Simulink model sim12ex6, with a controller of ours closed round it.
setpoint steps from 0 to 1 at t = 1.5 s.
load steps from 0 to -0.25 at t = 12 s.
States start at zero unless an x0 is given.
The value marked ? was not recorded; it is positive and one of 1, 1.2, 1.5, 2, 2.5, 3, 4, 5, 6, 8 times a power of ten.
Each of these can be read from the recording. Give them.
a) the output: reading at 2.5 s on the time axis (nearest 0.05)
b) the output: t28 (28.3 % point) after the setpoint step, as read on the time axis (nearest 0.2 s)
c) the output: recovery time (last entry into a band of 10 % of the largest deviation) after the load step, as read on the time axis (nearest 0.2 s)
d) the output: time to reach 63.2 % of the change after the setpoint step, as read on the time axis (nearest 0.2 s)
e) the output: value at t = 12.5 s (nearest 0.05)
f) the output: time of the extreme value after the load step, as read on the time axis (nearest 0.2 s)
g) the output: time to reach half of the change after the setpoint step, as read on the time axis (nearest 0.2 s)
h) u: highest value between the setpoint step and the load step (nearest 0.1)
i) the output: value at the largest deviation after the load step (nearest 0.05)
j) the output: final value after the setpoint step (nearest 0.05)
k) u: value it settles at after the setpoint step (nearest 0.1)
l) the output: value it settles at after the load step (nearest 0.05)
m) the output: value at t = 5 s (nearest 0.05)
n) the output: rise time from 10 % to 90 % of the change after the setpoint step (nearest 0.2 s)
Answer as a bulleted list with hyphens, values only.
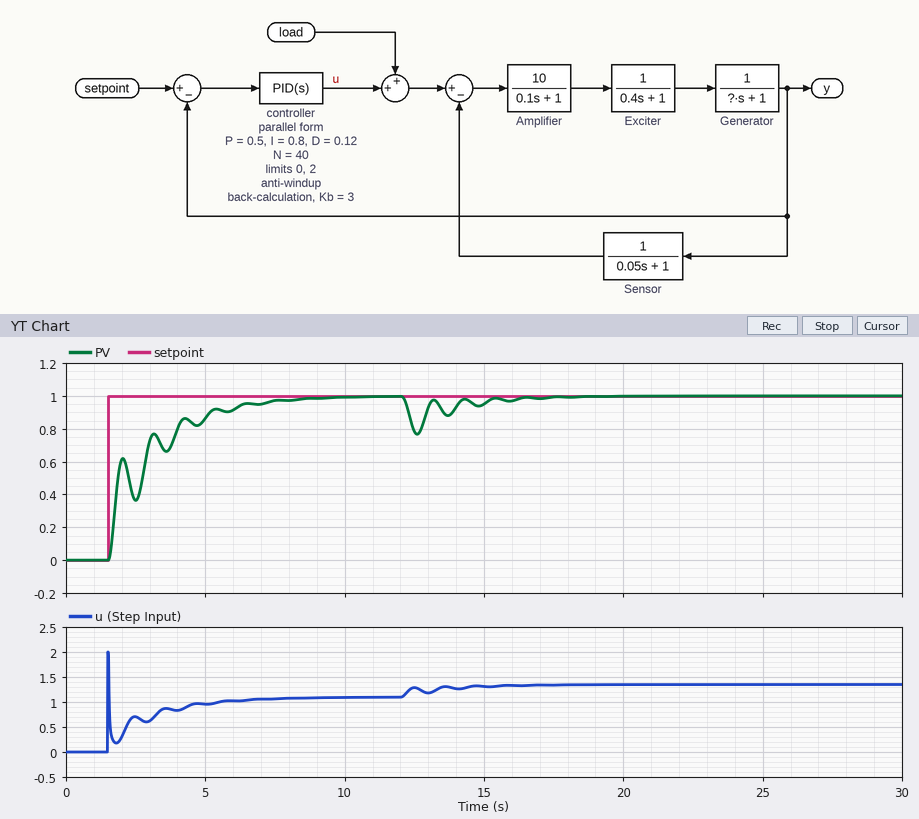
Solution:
- 0.35
- 1.8 s
- 16.2 s
- 2.8 s
- 0.80
- 12.6 s
- 1.8 s
- 2.0
- 0.75
- 1.00
- 1.1
- 1.00
- 0.85
- 3.6 s
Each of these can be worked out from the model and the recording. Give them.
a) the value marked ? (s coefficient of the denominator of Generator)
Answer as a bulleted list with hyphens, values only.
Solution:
- 1
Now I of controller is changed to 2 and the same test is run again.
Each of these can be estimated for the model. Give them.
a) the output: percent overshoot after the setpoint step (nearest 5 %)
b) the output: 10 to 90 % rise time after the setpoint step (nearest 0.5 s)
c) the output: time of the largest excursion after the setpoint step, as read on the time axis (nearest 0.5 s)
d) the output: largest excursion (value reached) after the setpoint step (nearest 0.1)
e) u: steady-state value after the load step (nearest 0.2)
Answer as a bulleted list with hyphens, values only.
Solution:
- 10 %
- 1.5 s
- 4.5 s
- 1.1
- 1.4
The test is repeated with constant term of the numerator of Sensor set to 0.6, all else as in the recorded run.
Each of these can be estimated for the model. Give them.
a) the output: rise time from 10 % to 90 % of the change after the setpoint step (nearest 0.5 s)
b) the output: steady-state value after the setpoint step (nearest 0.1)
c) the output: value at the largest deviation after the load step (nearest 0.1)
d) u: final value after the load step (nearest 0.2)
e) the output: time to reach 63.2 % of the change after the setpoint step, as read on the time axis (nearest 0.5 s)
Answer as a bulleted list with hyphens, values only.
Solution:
- 2.5 s
- 1.0
- 0.7
- 1.0
- 2.0 s
